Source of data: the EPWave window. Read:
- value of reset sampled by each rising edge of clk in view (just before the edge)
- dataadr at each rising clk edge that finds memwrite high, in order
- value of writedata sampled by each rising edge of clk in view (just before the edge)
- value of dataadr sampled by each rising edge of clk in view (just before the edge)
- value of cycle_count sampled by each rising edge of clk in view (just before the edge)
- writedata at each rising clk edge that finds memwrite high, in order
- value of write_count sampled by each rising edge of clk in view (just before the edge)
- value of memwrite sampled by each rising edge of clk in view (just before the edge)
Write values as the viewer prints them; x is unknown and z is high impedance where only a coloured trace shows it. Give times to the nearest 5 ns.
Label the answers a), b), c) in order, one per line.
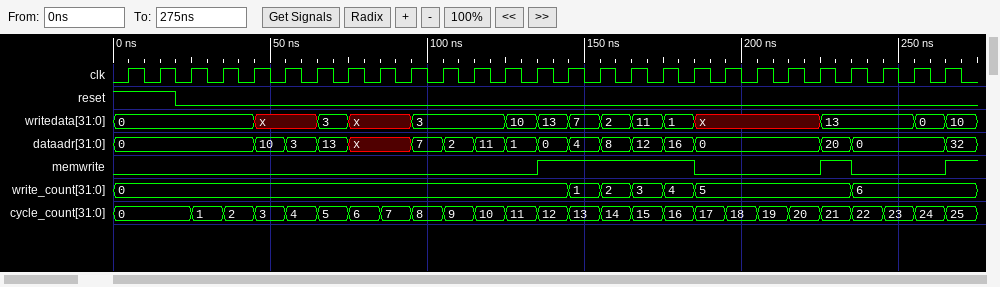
a) 1 1 0 0 0 0 0 0 0 0 0 0 0 0 0 0 0 0 0 0 0 0 0 0 0 0 0
b) 0, 4, 8, 12, 16, 20
c) 0, 0, 0, 0, 0, x, x, 3, x, x, 3, 3, 3, 10, 13, 7, 2, 11, 1, x, x, x, x, 13, 13, 13, 0
d) 0, 0, 0, 0, 0, 10, 3, 13, x, x, 7, 2, 11, 1, 0, 4, 8, 12, 16, 0, 0, 0, 0, 20, 0, 0, 0
e) 0, 0, 0, 1, 2, 3, 4, 5, 6, 7, 8, 9, 10, 11, 12, 13, 14, 15, 16, 17, 18, 19, 20, 21, 22, 23, 24
f) 13, 7, 2, 11, 1, 13
g) 0, 0, 0, 0, 0, 0, 0, 0, 0, 0, 0, 0, 0, 0, 0, 1, 2, 3, 4, 5, 5, 5, 5, 5, 6, 6, 6
h) 0 0 0 0 0 0 0 0 0 0 0 0 0 0 1 1 1 1 1 0 0 0 0 1 0 0 0
